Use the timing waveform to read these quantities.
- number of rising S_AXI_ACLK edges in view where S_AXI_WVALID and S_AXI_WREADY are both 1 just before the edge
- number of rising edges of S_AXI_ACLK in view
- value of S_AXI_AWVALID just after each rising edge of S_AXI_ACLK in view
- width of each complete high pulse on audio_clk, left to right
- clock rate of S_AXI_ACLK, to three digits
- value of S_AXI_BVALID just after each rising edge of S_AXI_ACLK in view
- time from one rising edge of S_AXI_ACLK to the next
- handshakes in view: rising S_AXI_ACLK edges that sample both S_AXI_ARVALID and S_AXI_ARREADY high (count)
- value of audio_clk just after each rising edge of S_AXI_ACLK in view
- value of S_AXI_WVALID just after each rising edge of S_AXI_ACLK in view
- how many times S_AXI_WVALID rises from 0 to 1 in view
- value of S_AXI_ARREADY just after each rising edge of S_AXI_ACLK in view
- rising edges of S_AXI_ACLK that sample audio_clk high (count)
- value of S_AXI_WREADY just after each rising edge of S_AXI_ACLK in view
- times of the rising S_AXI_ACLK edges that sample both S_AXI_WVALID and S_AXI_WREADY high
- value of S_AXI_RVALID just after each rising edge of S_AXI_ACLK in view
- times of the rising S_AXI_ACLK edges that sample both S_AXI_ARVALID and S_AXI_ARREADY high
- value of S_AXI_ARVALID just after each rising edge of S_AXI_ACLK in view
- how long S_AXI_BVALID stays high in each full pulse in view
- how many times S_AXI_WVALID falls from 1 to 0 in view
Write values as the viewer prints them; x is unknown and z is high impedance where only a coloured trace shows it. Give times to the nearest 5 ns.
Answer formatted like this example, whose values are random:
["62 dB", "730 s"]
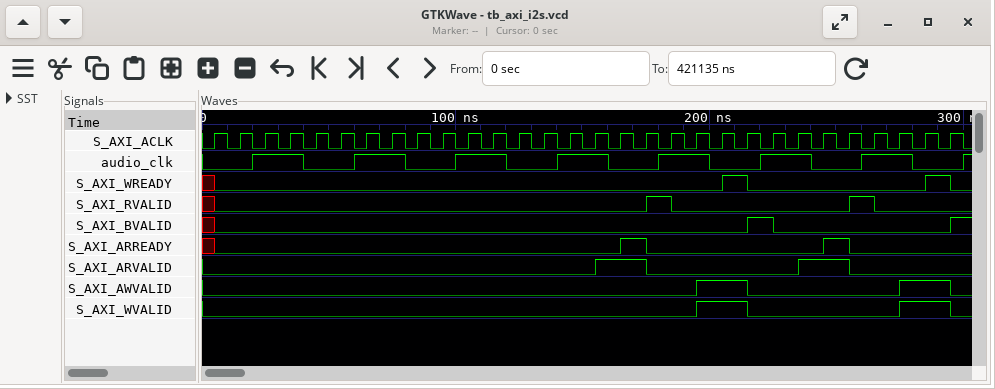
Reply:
["2", "30", "0 0 0 0 0 0 0 0 0 0 0 0 0 0 0 0 0 0 0 1 1 0 0 0 0 0 0 1 1 0", "20 ns, 20 ns, 20 ns, 20 ns, 20 ns, 20 ns, 20 ns", "100 MHz", "0 0 0 0 0 0 0 0 0 0 0 0 0 0 0 0 0 0 0 0 0 1 0 0 0 0 0 0 0 1", "10 ns", "2", "0 0 1 1 0 0 1 1 0 0 1 1 0 0 1 1 0 0 1 1 0 0 1 1 0 0 1 1 0 0", "0 0 0 0 0 0 0 0 0 0 0 0 0 0 0 0 0 0 0 1 1 0 0 0 0 0 0 1 1 0", "2", "0 0 0 0 0 0 0 0 0 0 0 0 0 0 0 0 1 0 0 0 0 0 0 0 1 0 0 0 0 0", "14", "0 0 0 0 0 0 0 0 0 0 0 0 0 0 0 0 0 0 0 0 1 0 0 0 0 0 0 0 1 0", "215 ns, 295 ns", "0 0 0 0 0 0 0 0 0 0 0 0 0 0 0 0 0 1 0 0 0 0 0 0 0 1 0 0 0 0", "175 ns, 255 ns", "0 0 0 0 0 0 0 0 0 0 0 0 0 0 0 1 1 0 0 0 0 0 0 1 1 0 0 0 0 0", "10 ns", "2"]
